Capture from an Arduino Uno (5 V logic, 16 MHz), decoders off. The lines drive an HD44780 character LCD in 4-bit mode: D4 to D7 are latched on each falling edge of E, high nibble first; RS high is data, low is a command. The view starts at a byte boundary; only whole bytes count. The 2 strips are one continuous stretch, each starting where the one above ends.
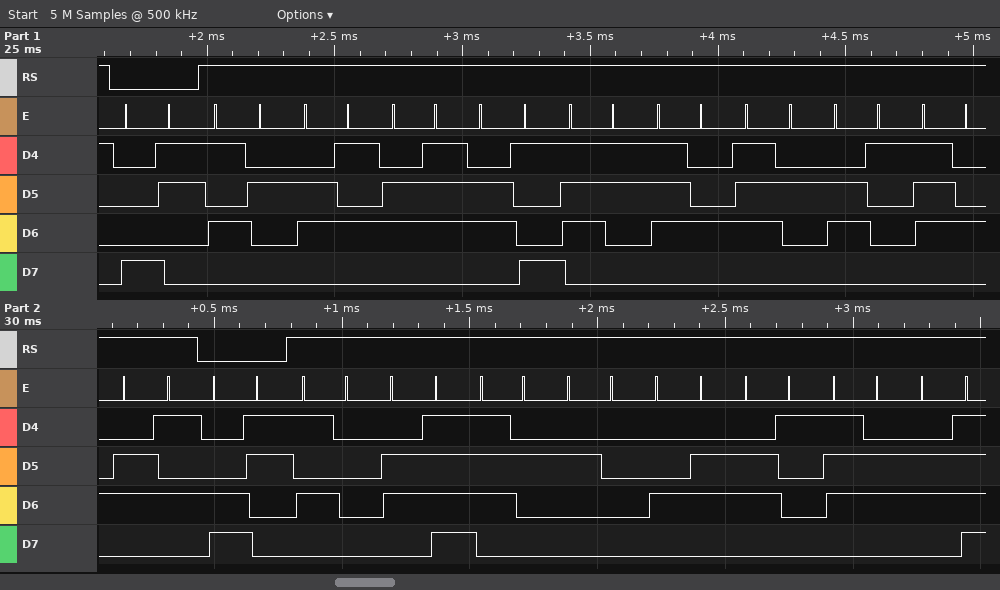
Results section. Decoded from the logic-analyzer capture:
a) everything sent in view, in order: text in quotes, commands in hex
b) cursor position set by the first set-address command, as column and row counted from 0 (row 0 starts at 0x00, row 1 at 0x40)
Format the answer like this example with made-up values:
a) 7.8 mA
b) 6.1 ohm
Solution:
a) 0x83 "Registrate" 0xC3 "Por Favo"
b) column 3, row 0
